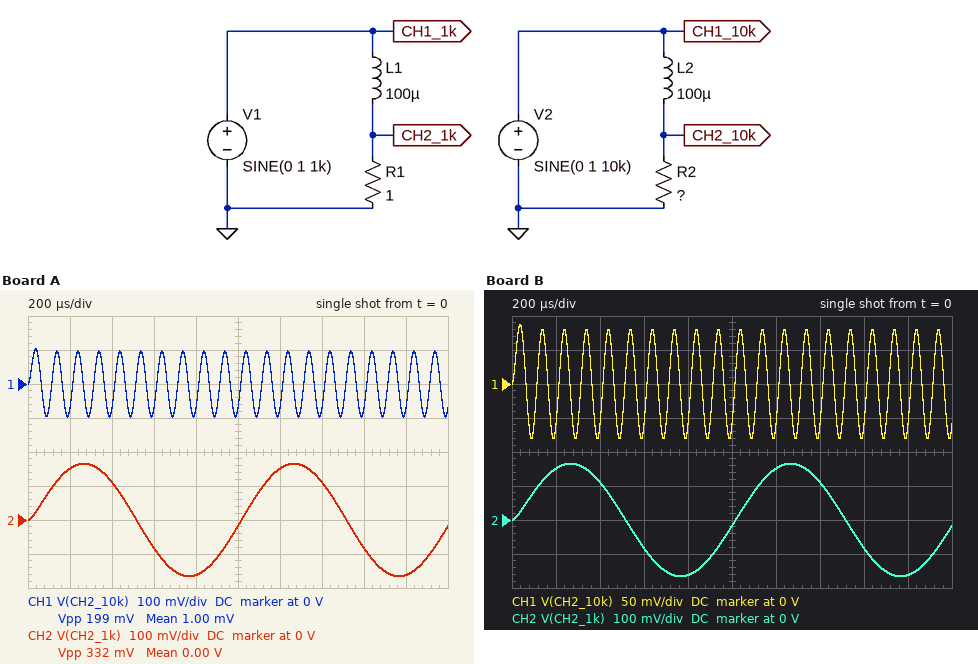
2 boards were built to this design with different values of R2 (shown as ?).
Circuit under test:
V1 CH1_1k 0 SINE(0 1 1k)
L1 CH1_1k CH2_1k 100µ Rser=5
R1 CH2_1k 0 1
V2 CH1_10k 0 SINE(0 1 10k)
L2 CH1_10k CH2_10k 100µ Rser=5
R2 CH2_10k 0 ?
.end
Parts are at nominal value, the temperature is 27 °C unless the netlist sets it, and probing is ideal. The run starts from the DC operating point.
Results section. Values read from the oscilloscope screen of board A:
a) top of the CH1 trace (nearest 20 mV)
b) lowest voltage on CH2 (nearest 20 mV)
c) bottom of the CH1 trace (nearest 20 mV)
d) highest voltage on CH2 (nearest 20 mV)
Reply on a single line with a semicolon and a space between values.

100 mV; -160 mV; -100 mV; 160 mV
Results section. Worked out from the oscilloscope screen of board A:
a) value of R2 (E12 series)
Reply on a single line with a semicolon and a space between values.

0.82 Ω
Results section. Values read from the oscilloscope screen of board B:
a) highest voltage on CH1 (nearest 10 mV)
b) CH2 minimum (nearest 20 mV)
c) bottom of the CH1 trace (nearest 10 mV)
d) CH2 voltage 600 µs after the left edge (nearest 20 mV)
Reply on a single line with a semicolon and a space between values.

90 mV; -160 mV; -80 mV; -80 mV
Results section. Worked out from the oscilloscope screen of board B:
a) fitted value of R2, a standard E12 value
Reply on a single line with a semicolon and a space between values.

0.68 Ω
